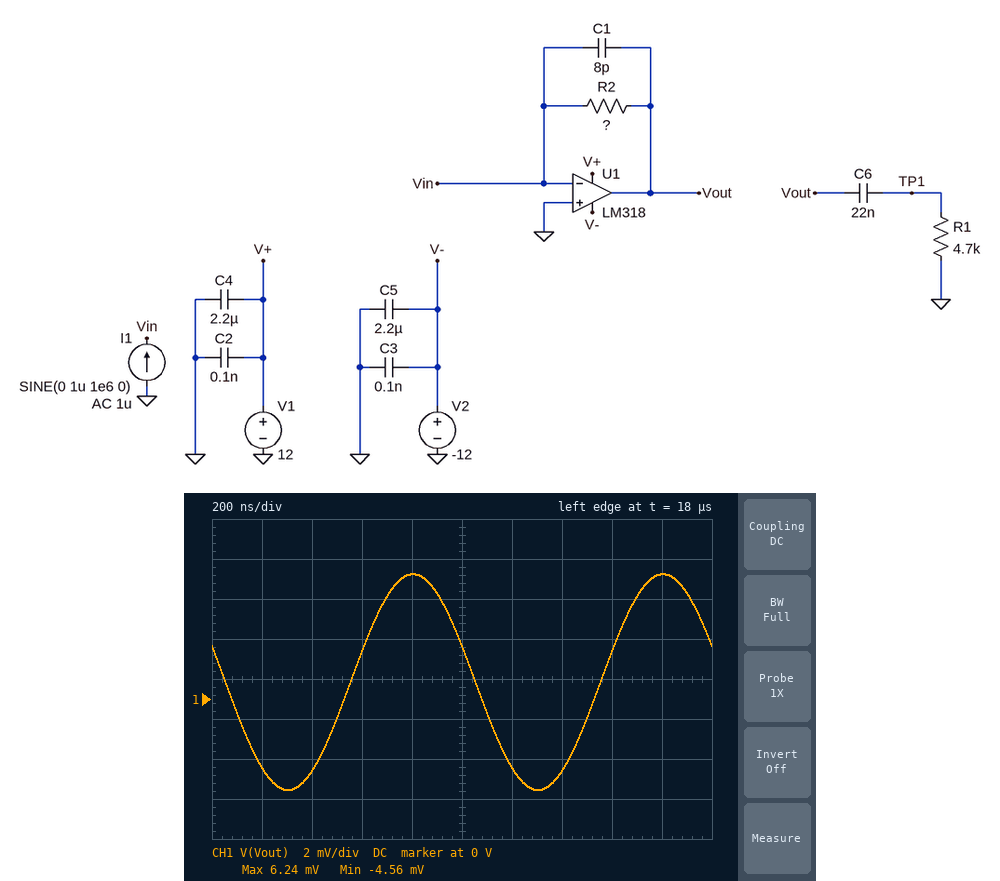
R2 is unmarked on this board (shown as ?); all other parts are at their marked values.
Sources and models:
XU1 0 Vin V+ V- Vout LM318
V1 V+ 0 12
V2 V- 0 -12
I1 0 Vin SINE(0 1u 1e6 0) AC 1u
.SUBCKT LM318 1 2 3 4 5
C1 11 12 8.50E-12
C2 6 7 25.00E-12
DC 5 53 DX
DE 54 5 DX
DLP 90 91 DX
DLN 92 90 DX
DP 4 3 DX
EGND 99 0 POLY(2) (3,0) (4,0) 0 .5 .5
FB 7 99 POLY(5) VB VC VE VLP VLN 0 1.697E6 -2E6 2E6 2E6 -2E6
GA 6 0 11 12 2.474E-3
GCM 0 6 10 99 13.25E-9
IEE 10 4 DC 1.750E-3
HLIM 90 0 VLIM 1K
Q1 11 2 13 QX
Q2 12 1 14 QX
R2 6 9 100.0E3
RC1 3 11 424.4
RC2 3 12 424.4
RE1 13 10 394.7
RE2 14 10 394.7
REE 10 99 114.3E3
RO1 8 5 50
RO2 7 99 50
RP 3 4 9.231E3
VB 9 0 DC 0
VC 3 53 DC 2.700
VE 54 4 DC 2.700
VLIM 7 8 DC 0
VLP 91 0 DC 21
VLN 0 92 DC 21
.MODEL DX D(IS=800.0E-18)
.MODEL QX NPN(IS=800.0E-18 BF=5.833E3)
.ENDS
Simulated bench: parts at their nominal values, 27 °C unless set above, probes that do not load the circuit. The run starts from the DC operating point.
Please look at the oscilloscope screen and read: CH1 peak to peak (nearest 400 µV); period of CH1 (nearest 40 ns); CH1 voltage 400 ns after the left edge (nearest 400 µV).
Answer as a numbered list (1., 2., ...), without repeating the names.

1. 10.8 mV
2. 1.00 µs
3. -3.6 mV
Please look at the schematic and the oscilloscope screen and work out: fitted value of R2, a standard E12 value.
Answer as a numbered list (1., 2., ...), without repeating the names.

1. 5.6 kΩ
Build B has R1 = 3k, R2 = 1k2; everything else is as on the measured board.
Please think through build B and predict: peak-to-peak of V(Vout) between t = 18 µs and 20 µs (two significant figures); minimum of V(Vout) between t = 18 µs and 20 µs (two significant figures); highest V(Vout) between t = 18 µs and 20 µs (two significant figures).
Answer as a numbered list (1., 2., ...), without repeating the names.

1. 2.4 mV
2. -1.0 mV
3. 1.4 mV
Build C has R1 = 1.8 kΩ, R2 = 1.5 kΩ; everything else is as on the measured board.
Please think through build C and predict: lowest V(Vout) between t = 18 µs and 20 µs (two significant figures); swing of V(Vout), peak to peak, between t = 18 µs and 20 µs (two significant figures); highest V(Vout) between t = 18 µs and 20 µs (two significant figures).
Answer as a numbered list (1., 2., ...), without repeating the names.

1. -1.3 mV
2. 3.0 mV
3. 1.7 mV
